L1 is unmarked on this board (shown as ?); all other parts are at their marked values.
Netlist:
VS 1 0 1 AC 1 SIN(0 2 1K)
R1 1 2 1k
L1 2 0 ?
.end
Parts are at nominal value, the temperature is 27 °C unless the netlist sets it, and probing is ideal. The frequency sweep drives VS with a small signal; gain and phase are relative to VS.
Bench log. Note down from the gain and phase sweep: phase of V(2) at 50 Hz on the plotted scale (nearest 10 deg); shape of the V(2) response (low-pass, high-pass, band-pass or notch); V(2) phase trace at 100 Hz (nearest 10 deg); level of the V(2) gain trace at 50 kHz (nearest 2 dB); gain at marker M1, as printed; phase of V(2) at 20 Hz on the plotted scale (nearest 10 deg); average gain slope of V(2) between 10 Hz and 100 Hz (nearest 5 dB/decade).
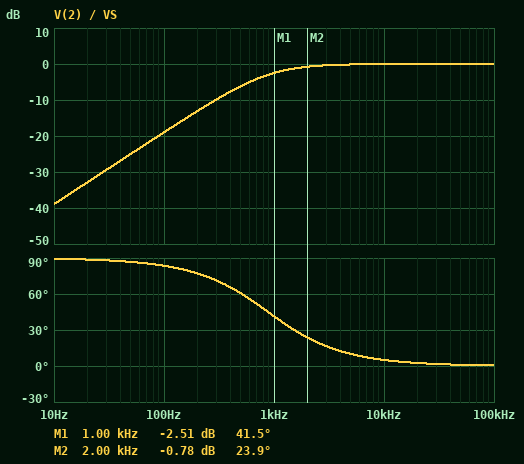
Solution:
90 deg
high-pass
80 deg
0 dB
-2.51 dB
90 deg
20 dB/decade
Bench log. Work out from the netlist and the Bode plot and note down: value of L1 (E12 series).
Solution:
180 mH
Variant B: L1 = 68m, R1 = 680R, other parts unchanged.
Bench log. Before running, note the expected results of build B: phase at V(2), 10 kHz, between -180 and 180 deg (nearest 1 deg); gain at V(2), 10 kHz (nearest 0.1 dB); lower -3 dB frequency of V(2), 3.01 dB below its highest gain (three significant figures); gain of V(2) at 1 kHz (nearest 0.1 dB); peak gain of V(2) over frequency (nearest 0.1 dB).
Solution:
9 deg
-0.1 dB
1.59 kHz
-5.5 dB
0 dB
